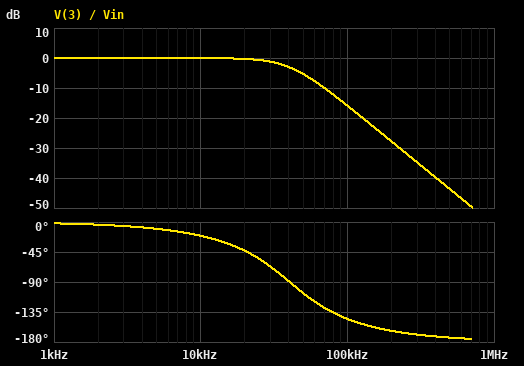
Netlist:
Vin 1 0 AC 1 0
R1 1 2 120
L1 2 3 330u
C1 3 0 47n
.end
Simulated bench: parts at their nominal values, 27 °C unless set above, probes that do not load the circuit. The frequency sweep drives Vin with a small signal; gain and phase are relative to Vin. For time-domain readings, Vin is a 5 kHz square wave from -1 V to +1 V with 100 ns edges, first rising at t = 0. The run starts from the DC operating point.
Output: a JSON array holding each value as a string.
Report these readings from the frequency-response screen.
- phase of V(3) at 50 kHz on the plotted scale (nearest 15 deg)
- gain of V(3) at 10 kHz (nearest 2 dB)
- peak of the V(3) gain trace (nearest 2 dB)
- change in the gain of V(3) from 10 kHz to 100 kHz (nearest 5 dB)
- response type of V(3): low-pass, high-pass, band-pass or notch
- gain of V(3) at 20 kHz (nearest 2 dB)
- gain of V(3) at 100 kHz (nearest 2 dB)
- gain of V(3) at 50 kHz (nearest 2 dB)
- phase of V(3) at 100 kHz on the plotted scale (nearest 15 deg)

["-105 deg", "0 dB", "0 dB", "-15 dB", "low-pass", "0 dB", "-16 dB", "-6 dB", "-150 deg"]
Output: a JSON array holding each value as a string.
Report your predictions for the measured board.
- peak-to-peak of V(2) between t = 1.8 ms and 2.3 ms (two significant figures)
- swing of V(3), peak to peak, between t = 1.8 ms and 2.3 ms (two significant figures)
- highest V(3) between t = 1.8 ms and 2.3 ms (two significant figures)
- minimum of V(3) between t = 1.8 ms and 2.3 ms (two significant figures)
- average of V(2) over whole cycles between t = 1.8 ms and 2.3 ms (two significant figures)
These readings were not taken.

["2.1 V", "2.2 V", "1.1 V", "-1.1 V", "170 mV"]
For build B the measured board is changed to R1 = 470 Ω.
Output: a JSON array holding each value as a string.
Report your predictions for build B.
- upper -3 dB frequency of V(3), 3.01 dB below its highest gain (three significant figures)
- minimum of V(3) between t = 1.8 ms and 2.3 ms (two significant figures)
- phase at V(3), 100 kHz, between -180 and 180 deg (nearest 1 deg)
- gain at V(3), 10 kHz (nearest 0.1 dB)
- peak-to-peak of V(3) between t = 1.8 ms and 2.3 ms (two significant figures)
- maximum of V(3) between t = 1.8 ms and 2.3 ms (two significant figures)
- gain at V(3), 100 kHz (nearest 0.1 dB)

["7.44 kHz", "-980 mV", "-110 deg", "-4.5 dB", "2.0 V", "980 mV", "-23.4 dB"]
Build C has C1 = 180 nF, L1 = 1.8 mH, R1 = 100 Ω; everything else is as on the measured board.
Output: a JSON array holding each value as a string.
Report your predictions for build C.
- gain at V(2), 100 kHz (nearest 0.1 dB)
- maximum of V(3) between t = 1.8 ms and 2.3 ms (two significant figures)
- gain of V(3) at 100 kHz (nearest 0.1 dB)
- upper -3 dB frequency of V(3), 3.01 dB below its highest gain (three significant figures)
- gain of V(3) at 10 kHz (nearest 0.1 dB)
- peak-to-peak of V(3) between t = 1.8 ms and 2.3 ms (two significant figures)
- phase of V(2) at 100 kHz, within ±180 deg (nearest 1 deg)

["0 dB", "1.3 V", "-42.1 dB", "10.3 kHz", "-1.3 dB", "2.7 V", "5 deg"]
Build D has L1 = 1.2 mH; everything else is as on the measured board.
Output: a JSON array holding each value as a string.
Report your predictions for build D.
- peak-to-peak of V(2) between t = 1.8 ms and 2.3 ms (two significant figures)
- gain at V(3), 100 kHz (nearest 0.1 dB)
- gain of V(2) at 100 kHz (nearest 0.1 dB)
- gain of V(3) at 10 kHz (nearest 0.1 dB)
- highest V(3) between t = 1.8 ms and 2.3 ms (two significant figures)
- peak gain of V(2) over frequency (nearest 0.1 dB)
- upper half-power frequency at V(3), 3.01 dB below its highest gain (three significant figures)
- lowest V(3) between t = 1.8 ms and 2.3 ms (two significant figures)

["2.5 V", "-26.7 dB", "-0.1 dB", "1.4 dB", "1.6 V", "0 dB", "25.2 kHz", "-1.6 V"]
